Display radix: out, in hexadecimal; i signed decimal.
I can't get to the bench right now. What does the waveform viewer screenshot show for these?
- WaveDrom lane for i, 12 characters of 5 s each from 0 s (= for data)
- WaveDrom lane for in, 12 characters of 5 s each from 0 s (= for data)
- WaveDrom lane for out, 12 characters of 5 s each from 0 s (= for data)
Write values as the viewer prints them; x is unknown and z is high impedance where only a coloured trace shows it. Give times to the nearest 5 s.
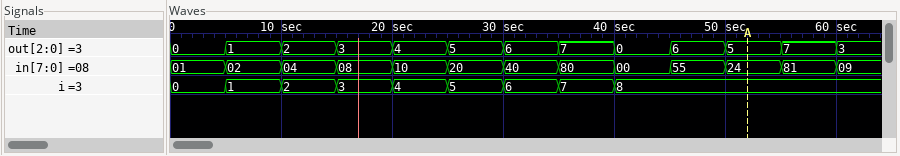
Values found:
{name: 'i', wave: '=========...', data: '0 1 2 3 4 5 6 7 8'}
{name: 'in', wave: '============', data: '01 02 04 08 10 20 40 80 00 55 24 81'}
{name: 'out', wave: '============', data: '0 1 2 3 4 5 6 7 0 6 5 7'}
